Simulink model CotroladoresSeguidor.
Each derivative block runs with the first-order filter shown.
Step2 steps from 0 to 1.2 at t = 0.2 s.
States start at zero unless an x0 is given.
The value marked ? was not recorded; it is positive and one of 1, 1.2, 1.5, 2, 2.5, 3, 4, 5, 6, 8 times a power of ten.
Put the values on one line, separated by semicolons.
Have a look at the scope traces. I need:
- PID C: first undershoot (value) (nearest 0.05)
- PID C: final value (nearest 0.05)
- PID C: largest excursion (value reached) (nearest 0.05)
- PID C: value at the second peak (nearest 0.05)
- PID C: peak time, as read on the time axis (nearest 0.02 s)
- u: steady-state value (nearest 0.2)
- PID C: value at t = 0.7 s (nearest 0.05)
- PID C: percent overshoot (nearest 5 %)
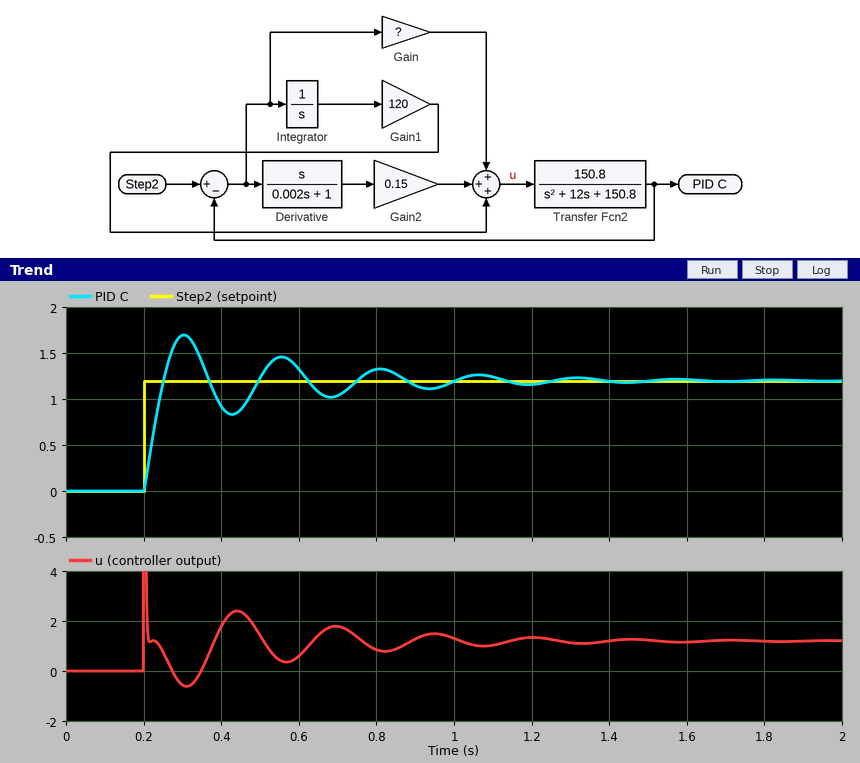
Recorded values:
0.85; 1.20; 1.70; 1.45; 0.30 s; 1.2; 1.05; 40 %
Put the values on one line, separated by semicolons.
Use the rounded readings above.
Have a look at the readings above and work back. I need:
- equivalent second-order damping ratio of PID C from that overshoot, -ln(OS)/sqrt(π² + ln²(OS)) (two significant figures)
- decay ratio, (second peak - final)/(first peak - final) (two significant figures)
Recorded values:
0.28; 0.50
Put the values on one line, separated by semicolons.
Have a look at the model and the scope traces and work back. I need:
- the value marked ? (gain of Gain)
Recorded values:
4
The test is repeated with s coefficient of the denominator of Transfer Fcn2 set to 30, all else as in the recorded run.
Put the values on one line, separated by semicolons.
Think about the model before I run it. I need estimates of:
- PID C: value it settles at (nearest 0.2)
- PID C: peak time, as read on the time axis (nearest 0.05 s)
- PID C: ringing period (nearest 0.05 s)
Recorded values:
1.2; 0.35 s; 0.30 s
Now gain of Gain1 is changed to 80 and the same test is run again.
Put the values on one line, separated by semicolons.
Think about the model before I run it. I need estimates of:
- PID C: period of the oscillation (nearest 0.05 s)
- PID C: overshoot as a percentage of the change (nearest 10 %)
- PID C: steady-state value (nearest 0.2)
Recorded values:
0.30 s; 30 %; 1.2
